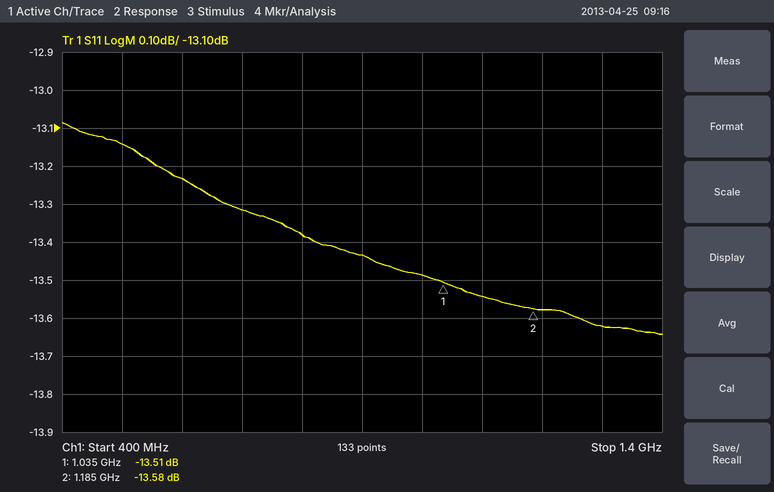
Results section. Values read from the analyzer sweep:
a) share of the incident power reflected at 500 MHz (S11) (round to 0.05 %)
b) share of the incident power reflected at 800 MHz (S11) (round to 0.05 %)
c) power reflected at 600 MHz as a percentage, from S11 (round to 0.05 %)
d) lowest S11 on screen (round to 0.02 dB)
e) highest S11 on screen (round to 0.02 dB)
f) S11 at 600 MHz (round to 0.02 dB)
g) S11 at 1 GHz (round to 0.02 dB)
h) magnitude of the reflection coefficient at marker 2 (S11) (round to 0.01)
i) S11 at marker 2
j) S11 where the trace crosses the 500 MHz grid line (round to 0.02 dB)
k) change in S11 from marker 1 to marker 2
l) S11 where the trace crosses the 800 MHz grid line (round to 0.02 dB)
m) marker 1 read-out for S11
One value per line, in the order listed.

4.85 %
4.60 %
4.75 %
-13.64 dB
-13.08 dB
-13.24 dB
-13.48 dB
0.21
-13.58 dB
-13.14 dB
-0.07 dB
-13.38 dB
-13.51 dB
